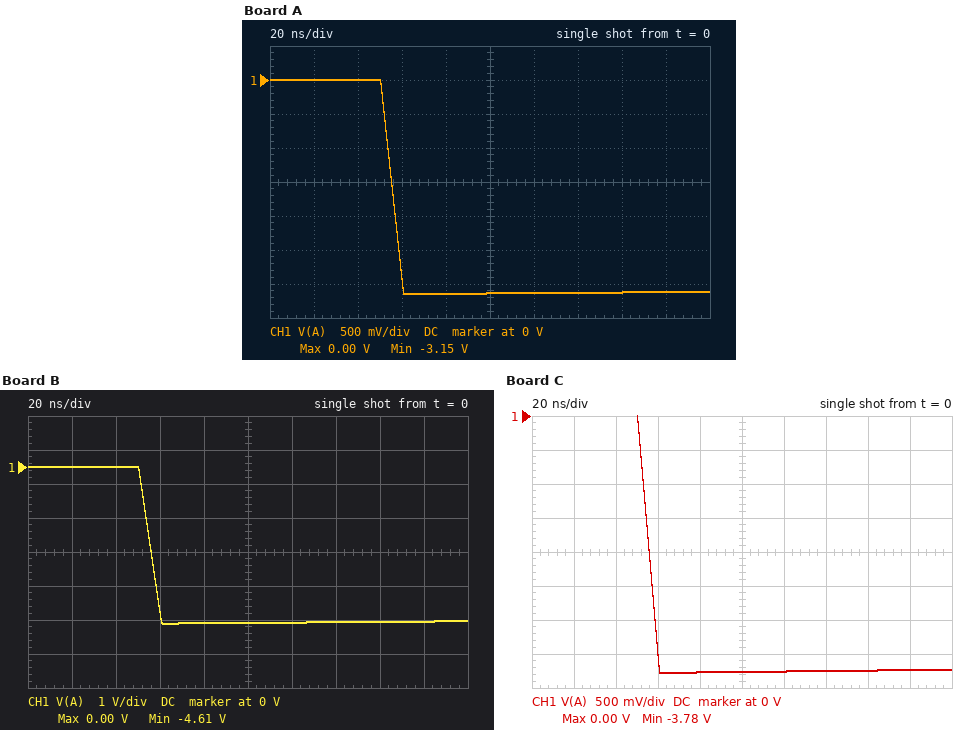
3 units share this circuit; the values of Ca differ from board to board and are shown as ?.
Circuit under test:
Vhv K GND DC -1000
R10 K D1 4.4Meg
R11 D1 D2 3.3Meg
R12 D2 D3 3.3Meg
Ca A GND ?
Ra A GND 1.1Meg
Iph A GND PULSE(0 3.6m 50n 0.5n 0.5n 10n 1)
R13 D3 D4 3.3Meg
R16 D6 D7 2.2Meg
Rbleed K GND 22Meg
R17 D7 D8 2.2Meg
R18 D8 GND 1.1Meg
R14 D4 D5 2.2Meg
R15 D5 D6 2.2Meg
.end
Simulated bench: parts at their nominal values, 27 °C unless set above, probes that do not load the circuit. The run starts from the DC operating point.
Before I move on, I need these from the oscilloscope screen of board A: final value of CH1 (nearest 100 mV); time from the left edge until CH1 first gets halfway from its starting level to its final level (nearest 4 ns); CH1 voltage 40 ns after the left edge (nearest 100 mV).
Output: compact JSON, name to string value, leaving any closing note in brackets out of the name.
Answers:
{"final value of CH1": "-3.1 V", "time from the left edge until CH1 first gets halfway from its starting level to its final level": "56 ns", "CH1 voltage 40 ns after the left edge": "0 V"}
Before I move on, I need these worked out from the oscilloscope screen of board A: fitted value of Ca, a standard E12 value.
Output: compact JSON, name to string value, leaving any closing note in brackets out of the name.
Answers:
{"fitted value of Ca, a standard E12 value": "12 pF"}
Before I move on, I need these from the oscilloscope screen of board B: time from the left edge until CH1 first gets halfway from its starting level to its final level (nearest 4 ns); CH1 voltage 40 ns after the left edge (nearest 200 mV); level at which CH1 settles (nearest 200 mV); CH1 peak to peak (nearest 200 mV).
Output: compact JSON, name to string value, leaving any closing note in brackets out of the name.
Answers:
{"time from the left edge until CH1 first gets halfway from its starting level to its final level": "56 ns", "CH1 voltage 40 ns after the left edge": "0 V", "level at which CH1 settles": "-4.6 V", "CH1 peak to peak": "4.6 V"}
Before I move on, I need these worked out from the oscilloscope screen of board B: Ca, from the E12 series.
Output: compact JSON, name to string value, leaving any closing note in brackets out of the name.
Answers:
{"Ca, from the E12 series": "8.2 pF"}
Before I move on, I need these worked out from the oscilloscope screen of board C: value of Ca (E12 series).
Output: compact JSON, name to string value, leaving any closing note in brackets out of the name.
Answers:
{"value of Ca": "10 pF"}
